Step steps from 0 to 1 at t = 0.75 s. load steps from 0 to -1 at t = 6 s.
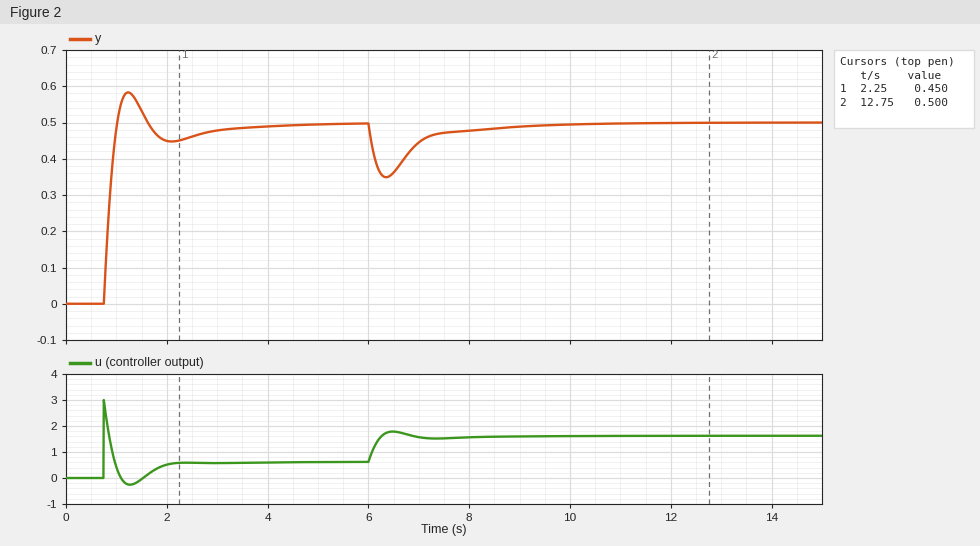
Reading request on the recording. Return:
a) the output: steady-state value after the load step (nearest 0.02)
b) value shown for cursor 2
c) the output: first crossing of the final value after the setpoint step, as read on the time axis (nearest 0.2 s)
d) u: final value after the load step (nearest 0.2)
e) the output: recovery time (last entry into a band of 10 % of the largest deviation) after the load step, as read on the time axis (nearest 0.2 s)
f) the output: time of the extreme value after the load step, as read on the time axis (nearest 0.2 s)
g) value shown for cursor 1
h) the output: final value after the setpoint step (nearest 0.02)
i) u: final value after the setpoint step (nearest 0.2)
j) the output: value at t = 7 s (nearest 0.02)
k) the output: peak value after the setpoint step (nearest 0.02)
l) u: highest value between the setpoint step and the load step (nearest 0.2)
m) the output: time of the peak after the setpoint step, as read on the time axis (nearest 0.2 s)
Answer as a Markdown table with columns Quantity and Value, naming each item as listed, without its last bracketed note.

| Quantity | Value |
|---|---|
| the output: steady-state value after the load step | 0.50 |
| value shown for cursor 2 | 0.500 |
| the output: first crossing of the final value after the setpoint step, as read on the time axis | 1.0 s |
| u: final value after the load step | 1.6 |
| the output: recovery time (last entry into a band of 10 % of the largest deviation) after the load step, as read on the time axis | 8.6 s |
| the output: time of the extreme value after the load step, as read on the time axis | 6.4 s |
| value shown for cursor 1 | 0.450 |
| the output: final value after the setpoint step | 0.50 |
| u: final value after the setpoint step | 0.6 |
| the output: value at t = 7 s | 0.44 |
| the output: peak value after the setpoint step | 0.58 |
| u: highest value between the setpoint step and the load step | 3.0 |
| the output: time of the peak after the setpoint step, as read on the time axis | 1.2 s |
